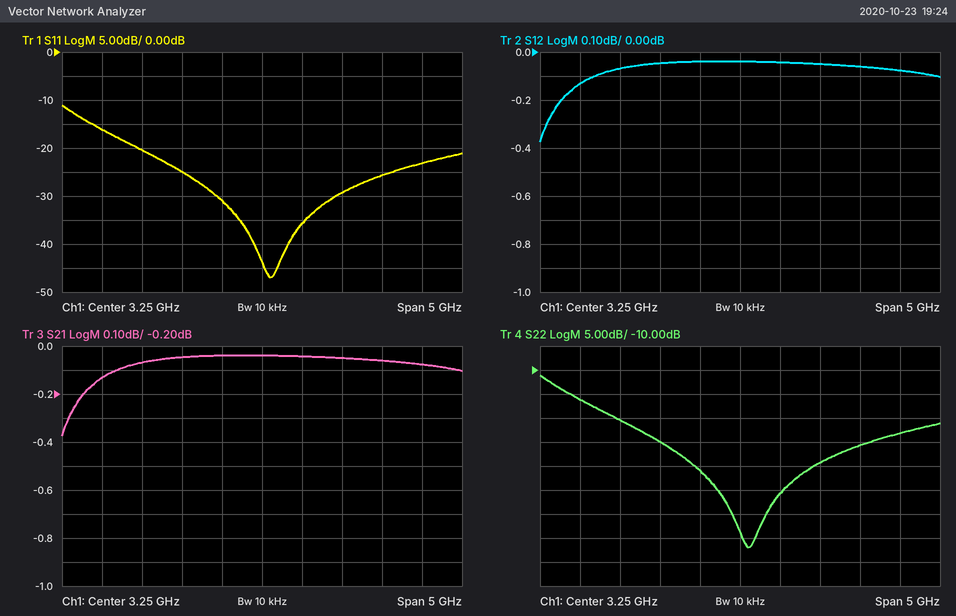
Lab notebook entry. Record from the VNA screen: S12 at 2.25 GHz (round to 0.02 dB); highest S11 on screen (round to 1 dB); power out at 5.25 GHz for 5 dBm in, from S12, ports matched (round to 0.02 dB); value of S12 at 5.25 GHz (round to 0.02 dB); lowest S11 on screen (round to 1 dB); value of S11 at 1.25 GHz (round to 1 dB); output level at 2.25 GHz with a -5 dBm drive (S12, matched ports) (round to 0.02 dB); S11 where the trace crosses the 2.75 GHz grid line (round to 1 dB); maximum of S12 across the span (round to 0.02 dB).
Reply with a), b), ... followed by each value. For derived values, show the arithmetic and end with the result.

a) -0.04 dB
b) -11 dB
c) 5 dBm + (-0.08 dB) = 4.92 dBm
d) -0.08 dB
e) -47 dB
f) -16 dB
g) -5 dBm + (-0.04 dB) = -5.04 dBm
h) -31 dB
i) -0.04 dB
